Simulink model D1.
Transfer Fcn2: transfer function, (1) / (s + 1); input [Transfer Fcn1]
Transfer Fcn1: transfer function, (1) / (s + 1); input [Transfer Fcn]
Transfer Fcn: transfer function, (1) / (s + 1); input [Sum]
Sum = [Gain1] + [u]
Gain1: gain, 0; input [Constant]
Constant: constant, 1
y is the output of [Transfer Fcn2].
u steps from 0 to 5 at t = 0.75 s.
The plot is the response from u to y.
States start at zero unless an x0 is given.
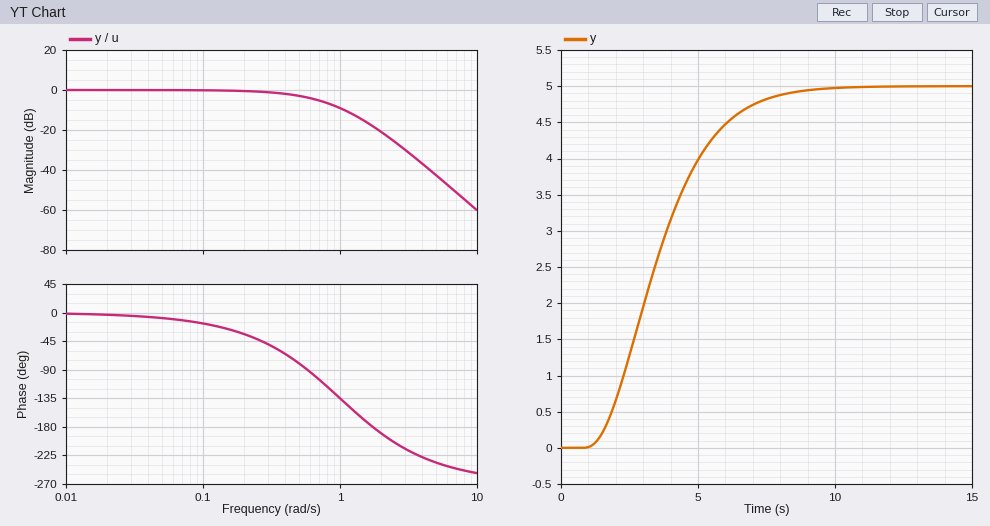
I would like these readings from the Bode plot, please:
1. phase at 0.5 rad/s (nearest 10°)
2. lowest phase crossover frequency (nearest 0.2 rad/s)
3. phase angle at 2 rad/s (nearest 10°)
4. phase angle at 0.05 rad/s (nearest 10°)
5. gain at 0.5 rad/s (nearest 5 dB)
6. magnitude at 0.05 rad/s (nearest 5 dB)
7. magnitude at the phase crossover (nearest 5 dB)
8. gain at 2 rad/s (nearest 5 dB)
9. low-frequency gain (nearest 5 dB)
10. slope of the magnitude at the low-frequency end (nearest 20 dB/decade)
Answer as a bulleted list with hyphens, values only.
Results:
- -80°
- 1.8 rad/s
- -190°
- -10°
- -5 dB
- 0 dB
- -20 dB
- -20 dB
- 0 dB
- 0 dB/decade
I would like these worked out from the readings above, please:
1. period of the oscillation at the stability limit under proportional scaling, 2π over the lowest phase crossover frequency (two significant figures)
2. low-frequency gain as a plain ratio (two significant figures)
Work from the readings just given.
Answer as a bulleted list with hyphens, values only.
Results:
- 3.5 s
- 1.0
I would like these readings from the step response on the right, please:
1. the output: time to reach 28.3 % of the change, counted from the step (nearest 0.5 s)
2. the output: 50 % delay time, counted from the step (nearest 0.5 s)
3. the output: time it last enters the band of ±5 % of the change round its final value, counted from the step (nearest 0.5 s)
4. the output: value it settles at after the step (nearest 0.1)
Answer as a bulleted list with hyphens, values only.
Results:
- 2.0 s
- 2.5 s
- 6.5 s
- 5.0
